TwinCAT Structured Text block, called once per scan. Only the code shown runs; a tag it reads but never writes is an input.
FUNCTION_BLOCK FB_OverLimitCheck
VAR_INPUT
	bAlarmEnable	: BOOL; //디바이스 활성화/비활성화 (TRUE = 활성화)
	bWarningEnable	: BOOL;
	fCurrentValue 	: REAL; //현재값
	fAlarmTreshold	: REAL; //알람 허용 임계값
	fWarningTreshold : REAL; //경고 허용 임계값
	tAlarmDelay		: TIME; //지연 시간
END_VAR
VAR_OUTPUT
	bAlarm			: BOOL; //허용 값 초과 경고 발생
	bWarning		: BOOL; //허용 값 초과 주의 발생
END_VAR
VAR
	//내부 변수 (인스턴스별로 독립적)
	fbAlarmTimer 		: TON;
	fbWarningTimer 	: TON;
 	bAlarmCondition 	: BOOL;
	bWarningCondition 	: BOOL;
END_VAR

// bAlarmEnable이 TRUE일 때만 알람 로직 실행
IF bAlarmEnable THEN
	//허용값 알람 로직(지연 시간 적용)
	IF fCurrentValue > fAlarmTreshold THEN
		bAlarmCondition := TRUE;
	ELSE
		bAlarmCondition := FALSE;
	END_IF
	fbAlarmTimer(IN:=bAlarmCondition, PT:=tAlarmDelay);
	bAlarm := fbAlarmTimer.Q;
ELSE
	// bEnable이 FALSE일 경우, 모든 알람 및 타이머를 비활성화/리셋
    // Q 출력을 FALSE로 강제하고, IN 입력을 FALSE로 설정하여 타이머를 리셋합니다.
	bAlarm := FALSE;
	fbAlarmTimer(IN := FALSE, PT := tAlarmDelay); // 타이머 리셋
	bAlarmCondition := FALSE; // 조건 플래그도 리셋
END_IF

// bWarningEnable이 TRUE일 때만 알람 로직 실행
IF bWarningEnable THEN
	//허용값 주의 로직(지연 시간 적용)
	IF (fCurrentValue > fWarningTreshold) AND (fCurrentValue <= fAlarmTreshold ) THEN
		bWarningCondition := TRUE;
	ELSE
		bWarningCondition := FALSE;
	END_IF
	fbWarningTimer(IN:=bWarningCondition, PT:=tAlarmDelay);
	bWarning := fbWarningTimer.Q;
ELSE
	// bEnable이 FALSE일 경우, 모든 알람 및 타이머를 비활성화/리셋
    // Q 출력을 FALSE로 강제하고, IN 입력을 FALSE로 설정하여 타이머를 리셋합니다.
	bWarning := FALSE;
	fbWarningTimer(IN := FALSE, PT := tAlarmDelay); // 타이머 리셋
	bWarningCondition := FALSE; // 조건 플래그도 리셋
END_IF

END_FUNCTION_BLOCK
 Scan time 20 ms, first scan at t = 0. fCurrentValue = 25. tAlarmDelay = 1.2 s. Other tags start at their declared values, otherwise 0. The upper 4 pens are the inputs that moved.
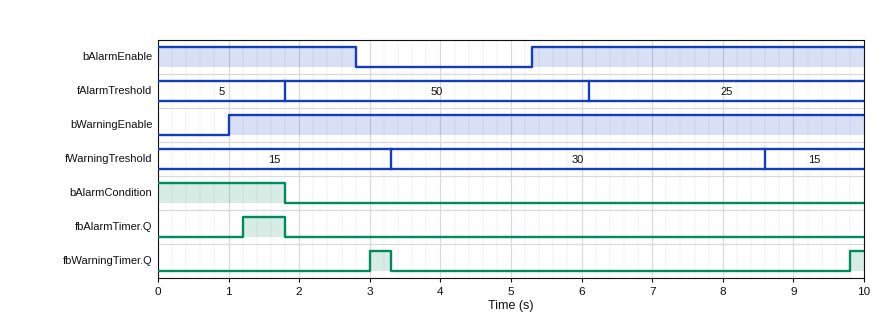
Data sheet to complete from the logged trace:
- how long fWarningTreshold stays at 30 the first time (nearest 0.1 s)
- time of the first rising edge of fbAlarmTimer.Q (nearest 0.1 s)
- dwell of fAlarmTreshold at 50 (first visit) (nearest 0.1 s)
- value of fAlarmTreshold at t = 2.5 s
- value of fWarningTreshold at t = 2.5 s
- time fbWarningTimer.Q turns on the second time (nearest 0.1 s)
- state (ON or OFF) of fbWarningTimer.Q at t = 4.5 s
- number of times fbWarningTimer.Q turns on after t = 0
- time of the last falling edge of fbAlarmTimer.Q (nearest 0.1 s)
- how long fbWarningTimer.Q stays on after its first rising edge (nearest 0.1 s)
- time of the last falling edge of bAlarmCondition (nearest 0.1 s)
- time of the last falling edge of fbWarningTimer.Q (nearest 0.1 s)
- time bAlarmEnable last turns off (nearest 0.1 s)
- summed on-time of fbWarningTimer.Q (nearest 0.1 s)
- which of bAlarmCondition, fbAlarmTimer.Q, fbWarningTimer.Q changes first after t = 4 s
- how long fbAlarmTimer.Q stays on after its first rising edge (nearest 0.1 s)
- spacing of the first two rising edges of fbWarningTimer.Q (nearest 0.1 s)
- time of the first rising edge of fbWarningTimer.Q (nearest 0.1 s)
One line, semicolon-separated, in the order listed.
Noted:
5.3 s; 1.2 s; 4.3 s; 50; 15; 9.8 s; OFF; 2; 1.8 s; 0.3 s; 1.8 s; 3.3 s; 2.8 s; 0.5 s; fbWarningTimer.Q; 0.6 s; 6.8 s; 3.0 s
